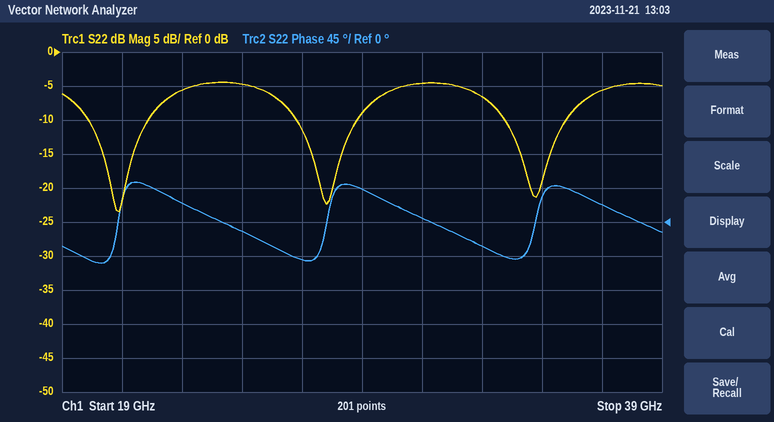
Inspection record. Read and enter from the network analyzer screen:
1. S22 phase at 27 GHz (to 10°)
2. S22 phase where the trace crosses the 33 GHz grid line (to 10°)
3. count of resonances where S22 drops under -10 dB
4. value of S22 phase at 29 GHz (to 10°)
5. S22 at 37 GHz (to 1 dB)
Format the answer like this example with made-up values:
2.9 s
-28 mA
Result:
-50°
-30°
3
40°
-6 dB
